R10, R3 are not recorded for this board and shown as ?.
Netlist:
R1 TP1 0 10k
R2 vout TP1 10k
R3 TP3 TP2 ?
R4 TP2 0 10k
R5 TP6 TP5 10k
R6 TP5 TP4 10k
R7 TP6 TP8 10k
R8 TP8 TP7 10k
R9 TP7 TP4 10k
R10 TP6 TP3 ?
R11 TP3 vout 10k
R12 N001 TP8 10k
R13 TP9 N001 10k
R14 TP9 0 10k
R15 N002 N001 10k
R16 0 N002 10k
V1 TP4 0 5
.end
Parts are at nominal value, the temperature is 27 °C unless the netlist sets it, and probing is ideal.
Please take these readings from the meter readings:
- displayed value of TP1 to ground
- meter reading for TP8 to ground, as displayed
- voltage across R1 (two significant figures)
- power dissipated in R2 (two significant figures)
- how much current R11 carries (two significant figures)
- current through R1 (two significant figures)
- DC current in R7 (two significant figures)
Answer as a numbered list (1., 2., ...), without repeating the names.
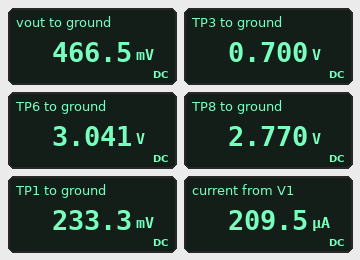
1. 233.3 mV
2. 2.770 V
3. 230 mV
4. 5.4 µW
5. 23 µA
6. 23 µA
7. 27 µA
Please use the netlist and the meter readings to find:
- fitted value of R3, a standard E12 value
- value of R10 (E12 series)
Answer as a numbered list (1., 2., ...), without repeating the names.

1. 4.7 kΩ
2. 33 kΩ
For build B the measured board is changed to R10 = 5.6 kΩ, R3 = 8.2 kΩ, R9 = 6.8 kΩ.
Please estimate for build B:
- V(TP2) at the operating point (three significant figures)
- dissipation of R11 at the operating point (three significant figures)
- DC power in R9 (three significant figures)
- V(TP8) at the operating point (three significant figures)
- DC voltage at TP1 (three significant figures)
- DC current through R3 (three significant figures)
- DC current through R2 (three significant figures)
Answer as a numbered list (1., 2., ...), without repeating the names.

1. 893 mV
2. 29.4 µW
3. 141 µW
4. 2.58 V
5. 542 mV
6. 89.3 µA
7. 54.2 µA
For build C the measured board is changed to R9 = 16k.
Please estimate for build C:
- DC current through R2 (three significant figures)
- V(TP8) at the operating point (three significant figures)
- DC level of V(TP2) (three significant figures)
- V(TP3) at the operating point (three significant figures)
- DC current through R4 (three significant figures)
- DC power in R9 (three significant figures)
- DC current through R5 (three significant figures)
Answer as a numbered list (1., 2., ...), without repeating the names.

1. 22.5 µA
2. 2.57 V
3. 458 mV
4. 674 mV
5. 45.8 µA
6. 139 µW
7. 104 µA
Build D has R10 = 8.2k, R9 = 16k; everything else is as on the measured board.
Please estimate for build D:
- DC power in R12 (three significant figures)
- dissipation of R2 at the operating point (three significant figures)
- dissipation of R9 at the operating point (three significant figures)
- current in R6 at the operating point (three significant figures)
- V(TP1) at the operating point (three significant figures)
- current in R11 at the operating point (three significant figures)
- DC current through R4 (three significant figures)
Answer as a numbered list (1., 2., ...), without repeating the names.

1. 126 µW
2. 17.7 µW
3. 179 µW
4. 134 µA
5. 421 mV
6. 42.1 µA
7. 85.9 µA
